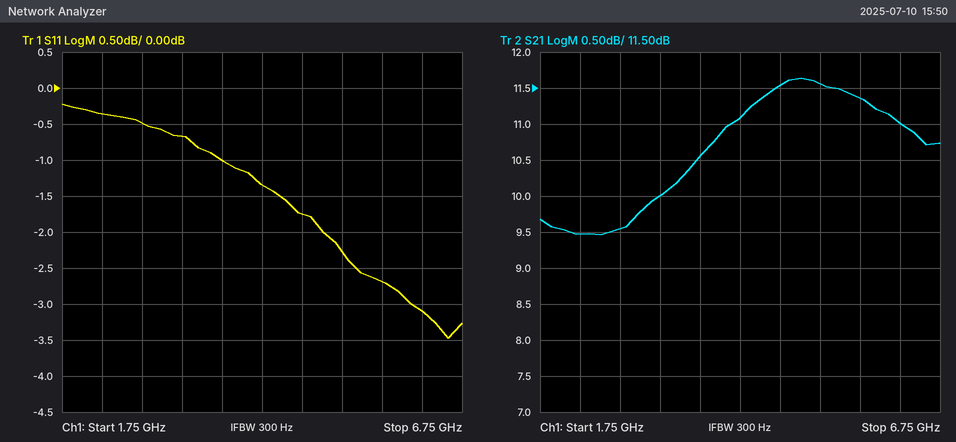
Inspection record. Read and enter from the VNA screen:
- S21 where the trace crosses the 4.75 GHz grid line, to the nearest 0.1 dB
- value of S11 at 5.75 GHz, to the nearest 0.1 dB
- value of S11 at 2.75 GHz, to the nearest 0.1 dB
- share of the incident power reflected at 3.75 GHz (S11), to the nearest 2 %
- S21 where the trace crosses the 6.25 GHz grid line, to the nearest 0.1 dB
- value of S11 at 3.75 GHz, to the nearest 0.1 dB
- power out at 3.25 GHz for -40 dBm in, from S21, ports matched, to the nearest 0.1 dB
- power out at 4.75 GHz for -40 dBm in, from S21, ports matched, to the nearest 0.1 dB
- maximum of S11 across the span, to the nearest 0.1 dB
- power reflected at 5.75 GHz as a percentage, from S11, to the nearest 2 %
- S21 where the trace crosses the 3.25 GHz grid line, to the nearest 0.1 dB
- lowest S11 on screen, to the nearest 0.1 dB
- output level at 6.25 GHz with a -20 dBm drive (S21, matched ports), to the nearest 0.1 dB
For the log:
11.5 dB
-2.7 dB
-0.5 dB
80 %
11.0 dB
-1.0 dB
-30.0 dBm
-28.5 dBm
-0.2 dB
54 %
10.0 dB
-3.5 dB
-9.0 dBm
